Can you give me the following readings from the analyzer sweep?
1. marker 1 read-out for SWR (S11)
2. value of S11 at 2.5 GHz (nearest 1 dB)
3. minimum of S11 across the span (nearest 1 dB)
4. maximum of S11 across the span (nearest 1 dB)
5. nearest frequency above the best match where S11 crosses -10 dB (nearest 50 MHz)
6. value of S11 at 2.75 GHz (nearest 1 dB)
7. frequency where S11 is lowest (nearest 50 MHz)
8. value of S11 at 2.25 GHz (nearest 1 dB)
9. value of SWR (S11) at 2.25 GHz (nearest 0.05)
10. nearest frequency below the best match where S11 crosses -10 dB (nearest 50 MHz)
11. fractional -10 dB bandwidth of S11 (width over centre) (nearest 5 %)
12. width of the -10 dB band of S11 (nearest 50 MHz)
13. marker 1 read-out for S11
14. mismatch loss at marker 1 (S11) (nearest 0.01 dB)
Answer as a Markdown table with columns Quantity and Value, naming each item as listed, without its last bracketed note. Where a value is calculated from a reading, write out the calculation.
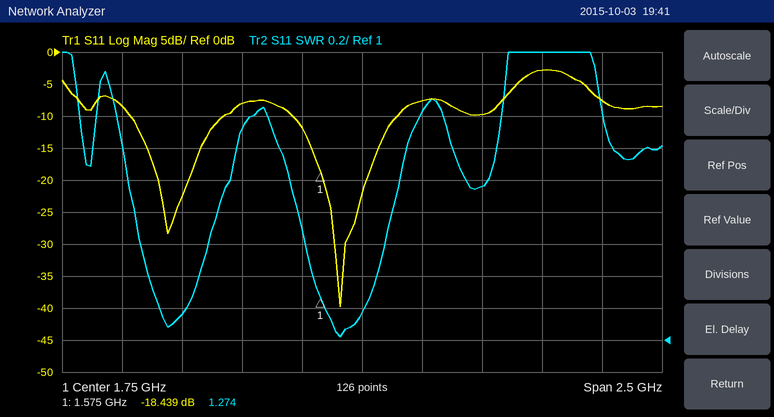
| Quantity | Value |
|---|---|
| marker 1 read-out for SWR | 1.274 |
| value of S11 at 2.5 GHz | -3 dB |
| minimum of S11 across the span | -40 dB |
| maximum of S11 across the span | -3 dB |
| nearest frequency above the best match where S11 crosses -10 dB | 1.90 GHz |
| value of S11 at 2.75 GHz | -8 dB |
| frequency where S11 is lowest | 1.65 GHz |
| value of S11 at 2.25 GHz | -10 dB |
| value of SWR (S11) at 2.25 GHz | 1.95 |
| nearest frequency below the best match where S11 crosses -10 dB | 1.45 GHz |
| fractional -10 dB bandwidth of S11 (width over centre) | 450 MHz / 1.675 GHz ≈ 26.9 %, so 25 % to the nearest 5 % |
| width of the -10 dB band of S11 | 1.90 GHz − 1.45 GHz = 450 MHz |
| marker 1 read-out for S11 | -18.439 dB |
| mismatch loss at marker 1 (S11) | −10 log10(1 − 10^(-18.439/10)) ≈ 0.06 dB |
